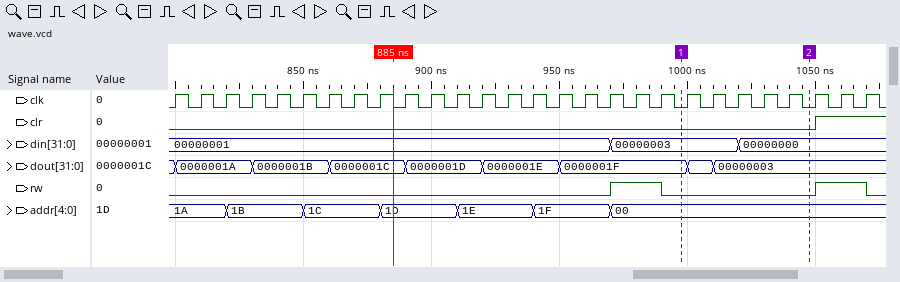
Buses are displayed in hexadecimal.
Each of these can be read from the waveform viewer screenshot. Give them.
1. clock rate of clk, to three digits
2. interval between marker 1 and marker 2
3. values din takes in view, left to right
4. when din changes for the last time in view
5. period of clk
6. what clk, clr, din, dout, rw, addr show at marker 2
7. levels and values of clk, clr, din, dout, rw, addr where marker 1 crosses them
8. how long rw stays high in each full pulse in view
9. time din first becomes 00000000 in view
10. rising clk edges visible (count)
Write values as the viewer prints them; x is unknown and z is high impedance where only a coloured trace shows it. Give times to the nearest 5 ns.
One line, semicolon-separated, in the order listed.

100 MHz; 50 ns; 00000001, 00000003, 00000000; 1020 ns; 10 ns; clk=0, clr=0, din=00000000, dout=00000003, rw=0, addr=00; clk=0, clr=0, din=00000003, dout=0000001F, rw=0, addr=00; 20 ns, 20 ns; 1020 ns; 28
